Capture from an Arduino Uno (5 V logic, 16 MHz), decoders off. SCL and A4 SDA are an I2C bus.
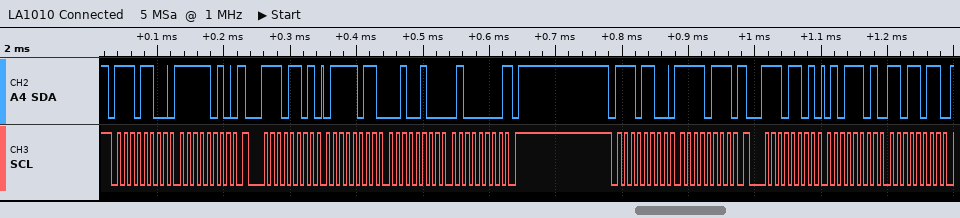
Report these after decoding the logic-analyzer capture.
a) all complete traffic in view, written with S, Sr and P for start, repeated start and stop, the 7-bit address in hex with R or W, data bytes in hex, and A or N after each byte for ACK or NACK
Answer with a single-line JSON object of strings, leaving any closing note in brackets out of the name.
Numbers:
{"all complete traffic in view, written with S, Sr and P for start, repeated start and stop, the 7-bit address in hex with R or W, data bytes in hex, and A or N after each byte for ACK or NACK": "S 76W A FA A Sr 76R A 7B A 24 A 40 N P S 76W A F7 A Sr 76R A 5D A DB A"}
